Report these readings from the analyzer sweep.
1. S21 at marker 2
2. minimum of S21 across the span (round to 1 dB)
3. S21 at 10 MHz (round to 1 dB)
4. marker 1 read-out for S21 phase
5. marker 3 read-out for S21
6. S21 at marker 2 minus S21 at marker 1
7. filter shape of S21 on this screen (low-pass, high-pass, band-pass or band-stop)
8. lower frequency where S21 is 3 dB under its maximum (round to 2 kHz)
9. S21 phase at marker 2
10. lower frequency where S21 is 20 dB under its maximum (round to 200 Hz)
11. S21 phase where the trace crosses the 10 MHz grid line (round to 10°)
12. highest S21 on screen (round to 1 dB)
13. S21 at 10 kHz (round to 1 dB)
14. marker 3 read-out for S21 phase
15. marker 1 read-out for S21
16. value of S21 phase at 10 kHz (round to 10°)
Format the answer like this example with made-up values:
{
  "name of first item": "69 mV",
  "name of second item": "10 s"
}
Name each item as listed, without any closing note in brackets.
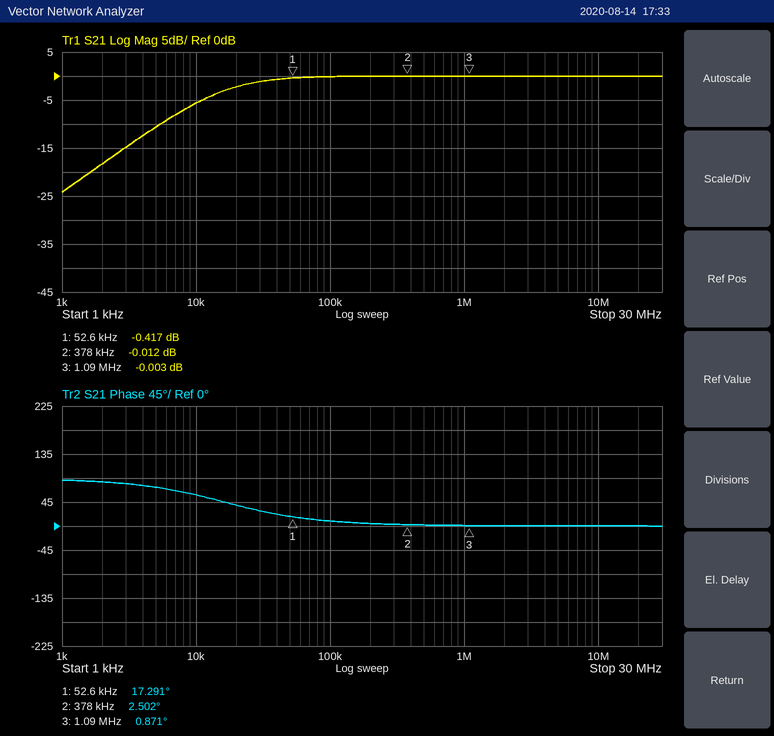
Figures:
{
  "S21 at marker 2": "-0.012 dB",
  "minimum of S21 across the span": "-24 dB",
  "S21 at 10 MHz": "0 dB",
  "marker 1 read-out for S21 phase": "17.291°",
  "marker 3 read-out for S21": "-0.003 dB",
  "S21 at marker 2 minus S21 at marker 1": "0.405 dB",
  "filter shape of S21 on this screen": "high-pass",
  "lower frequency where S21 is 3 dB under its maximum": "16 kHz",
  "S21 phase at marker 2": "2.502°",
  "lower frequency where S21 is 20 dB under its maximum": "1.6 kHz",
  "S21 phase where the trace crosses the 10 MHz grid line": "0°",
  "highest S21 on screen": "0 dB",
  "S21 at 10 kHz": "-6 dB",
  "marker 3 read-out for S21 phase": "0.871°",
  "marker 1 read-out for S21": "-0.417 dB",
  "value of S21 phase at 10 kHz": "60°"
}
